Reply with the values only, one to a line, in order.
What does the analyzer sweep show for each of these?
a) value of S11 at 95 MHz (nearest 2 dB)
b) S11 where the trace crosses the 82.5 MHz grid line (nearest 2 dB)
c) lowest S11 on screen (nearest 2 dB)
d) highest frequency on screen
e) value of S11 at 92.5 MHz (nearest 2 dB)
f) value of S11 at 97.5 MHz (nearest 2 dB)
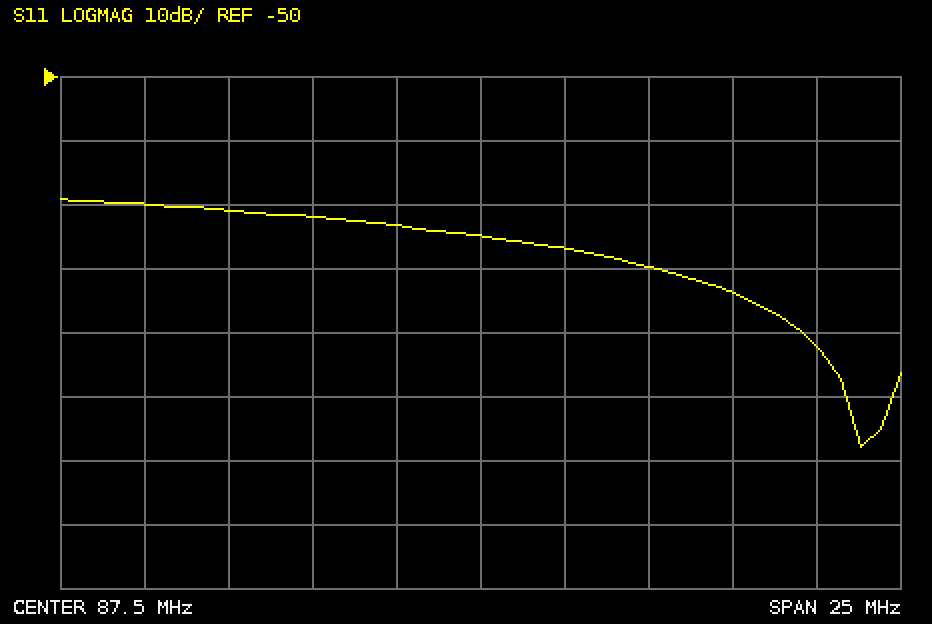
-84 dB
-72 dB
-108 dB
100 MHz
-80 dB
-92 dB
